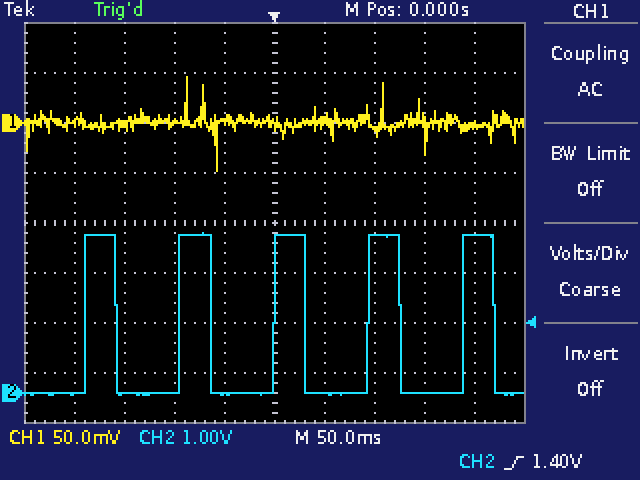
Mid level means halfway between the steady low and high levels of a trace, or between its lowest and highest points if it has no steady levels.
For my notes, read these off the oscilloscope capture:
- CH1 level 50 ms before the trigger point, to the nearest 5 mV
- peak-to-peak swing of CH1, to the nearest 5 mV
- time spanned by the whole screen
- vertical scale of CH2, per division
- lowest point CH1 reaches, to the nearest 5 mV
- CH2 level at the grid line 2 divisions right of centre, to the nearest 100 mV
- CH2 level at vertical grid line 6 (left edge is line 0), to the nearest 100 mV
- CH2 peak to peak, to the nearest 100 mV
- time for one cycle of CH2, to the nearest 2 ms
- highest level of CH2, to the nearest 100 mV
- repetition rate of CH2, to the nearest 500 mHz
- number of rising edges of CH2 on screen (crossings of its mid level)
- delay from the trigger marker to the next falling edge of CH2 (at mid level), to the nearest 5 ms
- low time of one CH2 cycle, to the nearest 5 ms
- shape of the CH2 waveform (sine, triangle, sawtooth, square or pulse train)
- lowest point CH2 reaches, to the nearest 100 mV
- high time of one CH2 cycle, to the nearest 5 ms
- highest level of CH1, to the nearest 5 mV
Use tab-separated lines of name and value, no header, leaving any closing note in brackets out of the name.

CH1 level 50 ms before the trigger point, to the nearest 5 mV	5 mV
peak-to-peak swing of CH1, to the nearest 5 mV	95 mV
time spanned by the whole screen	500 ms
vertical scale of CH2, per division	1 V
lowest point CH1 reaches, to the nearest 5 mV	-50 mV
CH2 level at the grid line 2 divisions right of centre, to the nearest 100 mV	3.2 V
CH2 level at vertical grid line 6 (left edge is line 0), to the nearest 100 mV	0.0 V
CH2 peak to peak, to the nearest 100 mV	3.2 V
time for one cycle of CH2, to the nearest 2 ms	94 ms
highest level of CH2, to the nearest 100 mV	3.2 V
repetition rate of CH2, to the nearest 500 mHz	10.5 Hz
number of rising edges of CH2 on screen	5
delay from the trigger marker to the next falling edge of CH2 (at mid level), to the nearest 5 ms	30 ms
low time of one CH2 cycle, to the nearest 5 ms	65 ms
shape of the CH2 waveform	pulse train
lowest point CH2 reaches, to the nearest 100 mV	0.0 V
high time of one CH2 cycle, to the nearest 5 ms	30 ms
highest level of CH1, to the nearest 5 mV	45 mV
